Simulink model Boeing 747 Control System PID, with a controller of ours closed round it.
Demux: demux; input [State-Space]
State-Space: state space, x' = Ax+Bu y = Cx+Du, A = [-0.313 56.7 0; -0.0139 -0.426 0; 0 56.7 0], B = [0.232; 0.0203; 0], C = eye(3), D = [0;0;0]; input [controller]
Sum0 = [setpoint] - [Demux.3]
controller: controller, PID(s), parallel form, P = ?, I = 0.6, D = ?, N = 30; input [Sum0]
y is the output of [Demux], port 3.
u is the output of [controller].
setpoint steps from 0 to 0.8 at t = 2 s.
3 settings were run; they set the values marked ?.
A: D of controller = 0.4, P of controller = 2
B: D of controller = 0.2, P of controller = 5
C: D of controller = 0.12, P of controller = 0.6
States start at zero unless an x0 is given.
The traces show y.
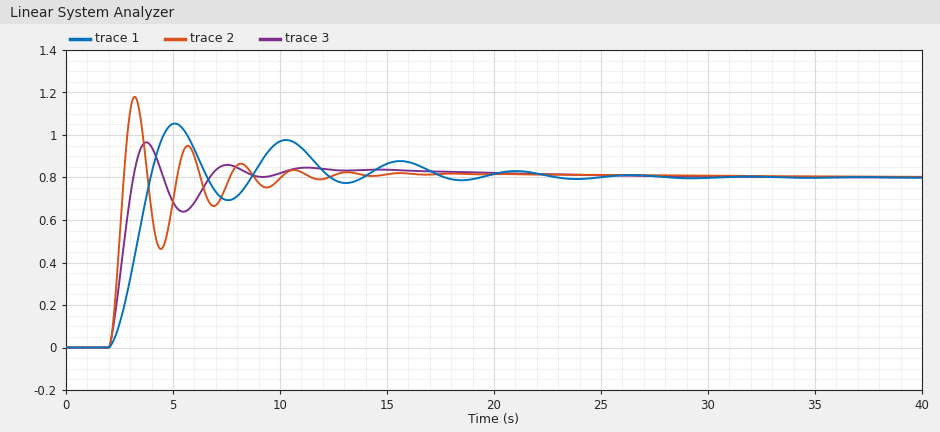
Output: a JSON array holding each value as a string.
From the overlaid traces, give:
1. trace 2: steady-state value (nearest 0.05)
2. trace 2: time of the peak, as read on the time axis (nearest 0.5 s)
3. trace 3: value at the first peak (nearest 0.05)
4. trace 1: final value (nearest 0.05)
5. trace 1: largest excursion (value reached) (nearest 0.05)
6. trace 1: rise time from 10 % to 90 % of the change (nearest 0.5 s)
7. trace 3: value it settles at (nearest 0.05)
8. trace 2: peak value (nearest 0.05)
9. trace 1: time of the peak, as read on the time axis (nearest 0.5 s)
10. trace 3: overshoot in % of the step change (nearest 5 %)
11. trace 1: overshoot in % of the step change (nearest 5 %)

["0.80", "3.0 s", "0.95", "0.80", "1.05", "1.5 s", "0.80", "1.20", "5.0 s", "20 %", "30 %"]
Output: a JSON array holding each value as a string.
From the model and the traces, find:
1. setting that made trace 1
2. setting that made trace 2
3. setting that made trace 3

["C", "B", "A"]
